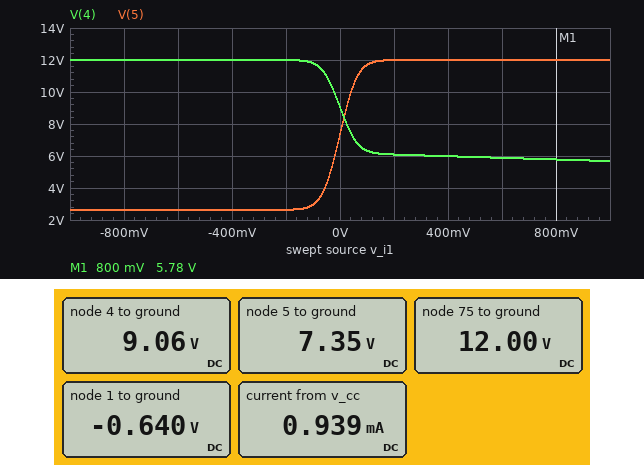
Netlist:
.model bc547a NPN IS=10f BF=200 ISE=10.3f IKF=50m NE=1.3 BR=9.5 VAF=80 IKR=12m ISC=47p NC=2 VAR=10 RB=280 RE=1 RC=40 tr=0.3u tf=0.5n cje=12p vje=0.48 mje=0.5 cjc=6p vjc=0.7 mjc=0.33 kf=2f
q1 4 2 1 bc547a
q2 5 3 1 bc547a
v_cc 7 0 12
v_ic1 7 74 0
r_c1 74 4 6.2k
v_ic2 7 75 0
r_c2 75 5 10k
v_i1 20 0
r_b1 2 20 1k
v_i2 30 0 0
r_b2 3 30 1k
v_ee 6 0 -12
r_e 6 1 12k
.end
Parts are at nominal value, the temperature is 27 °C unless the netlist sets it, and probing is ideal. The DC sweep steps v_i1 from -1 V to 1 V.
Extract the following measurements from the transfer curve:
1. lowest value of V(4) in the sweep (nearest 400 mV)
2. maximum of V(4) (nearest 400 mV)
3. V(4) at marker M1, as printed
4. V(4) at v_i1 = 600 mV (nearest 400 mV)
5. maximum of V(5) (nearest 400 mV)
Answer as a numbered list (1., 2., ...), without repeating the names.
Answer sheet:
1. 5.6 V
2. 12.0 V
3. 5.78 V
4. 6.0 V
5. 12.0 V
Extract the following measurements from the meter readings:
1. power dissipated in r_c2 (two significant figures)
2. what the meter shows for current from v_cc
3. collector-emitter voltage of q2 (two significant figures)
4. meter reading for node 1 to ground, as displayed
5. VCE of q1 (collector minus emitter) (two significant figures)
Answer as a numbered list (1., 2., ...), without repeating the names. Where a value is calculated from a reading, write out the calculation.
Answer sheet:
1. (12 V - 7.35 V)^2 / 10 kΩ = 2.2 mW
2. 0.939 mA
3. 7.35 V - (-640 mV) = 8.0 V
4. -0.640 V
5. 9.06 V - (-640 mV) = 9.7 V
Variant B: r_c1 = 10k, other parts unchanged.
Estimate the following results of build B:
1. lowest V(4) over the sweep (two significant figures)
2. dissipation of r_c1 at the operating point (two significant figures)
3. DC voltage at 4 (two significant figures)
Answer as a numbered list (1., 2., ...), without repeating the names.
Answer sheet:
1. 1.8 V
2. 2.2 mW
3. 7.3 V
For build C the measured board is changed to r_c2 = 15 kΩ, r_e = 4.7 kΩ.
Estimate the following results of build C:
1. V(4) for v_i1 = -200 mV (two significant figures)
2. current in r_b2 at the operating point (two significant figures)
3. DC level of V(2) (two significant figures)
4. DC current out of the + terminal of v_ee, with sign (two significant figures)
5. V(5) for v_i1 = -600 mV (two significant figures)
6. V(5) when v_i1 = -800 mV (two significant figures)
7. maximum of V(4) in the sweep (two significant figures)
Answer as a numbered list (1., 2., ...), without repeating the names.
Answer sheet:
1. 3.7 V
2. 22 µA
3. -13 mV
4. -2.4 mA
5. -1.2 V
6. -1.4 V
7. 8.5 V
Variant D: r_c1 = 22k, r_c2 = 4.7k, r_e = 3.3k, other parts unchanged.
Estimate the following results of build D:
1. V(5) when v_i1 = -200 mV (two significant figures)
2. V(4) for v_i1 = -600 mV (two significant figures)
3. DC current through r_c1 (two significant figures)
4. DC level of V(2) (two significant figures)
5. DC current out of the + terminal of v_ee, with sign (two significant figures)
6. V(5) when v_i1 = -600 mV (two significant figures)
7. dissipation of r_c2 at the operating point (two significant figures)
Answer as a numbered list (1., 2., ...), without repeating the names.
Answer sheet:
1. -690 mV
2. 9.5 V
3. 580 µA
4. -83 mV
5. -3.4 mA
6. -1.1 V
7. 34 mW
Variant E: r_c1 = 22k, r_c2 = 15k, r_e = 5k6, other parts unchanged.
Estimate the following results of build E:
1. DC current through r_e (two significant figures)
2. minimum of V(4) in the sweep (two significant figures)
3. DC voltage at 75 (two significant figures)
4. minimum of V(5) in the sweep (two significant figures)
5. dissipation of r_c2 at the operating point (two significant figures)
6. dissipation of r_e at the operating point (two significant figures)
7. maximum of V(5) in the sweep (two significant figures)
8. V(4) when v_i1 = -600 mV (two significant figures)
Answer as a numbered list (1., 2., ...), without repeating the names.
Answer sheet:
1. 2.0 mA
2. -1.2 V
3. 12 V
4. -1.6 V
5. 11 mW
6. 22 mW
7. 1.4 V
8. -1.1 V
